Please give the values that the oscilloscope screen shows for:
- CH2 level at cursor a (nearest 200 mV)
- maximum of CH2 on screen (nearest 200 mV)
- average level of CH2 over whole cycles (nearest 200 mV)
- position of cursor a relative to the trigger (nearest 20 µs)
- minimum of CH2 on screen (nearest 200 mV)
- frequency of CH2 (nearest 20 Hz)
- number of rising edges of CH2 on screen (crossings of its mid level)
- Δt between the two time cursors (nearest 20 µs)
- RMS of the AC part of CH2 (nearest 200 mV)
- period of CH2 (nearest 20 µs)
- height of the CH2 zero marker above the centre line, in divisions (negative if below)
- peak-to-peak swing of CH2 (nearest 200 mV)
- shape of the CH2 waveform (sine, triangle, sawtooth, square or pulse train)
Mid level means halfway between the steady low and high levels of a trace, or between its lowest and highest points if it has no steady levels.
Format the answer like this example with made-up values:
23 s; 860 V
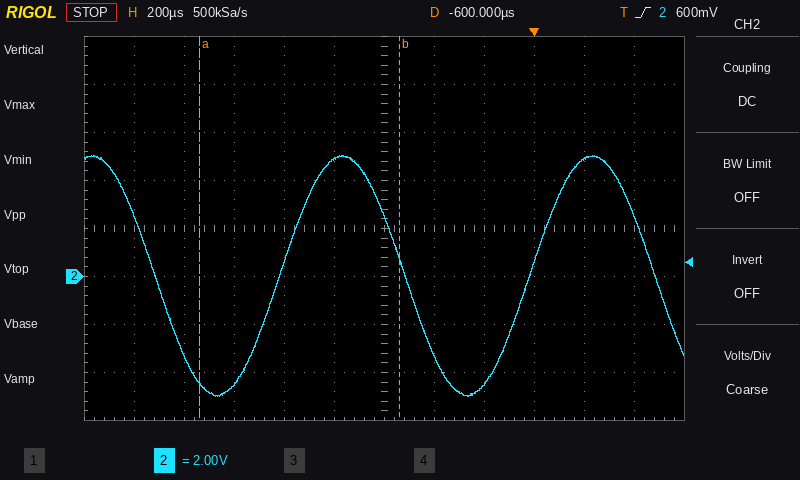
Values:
-4.4 V; 5.0 V; 0.0 V; -1.34 ms; -5.0 V; 1.00 kHz; 2; 800 µs; 3.6 V; 1.00 ms; -1.0 div; 10.0 V; sine
